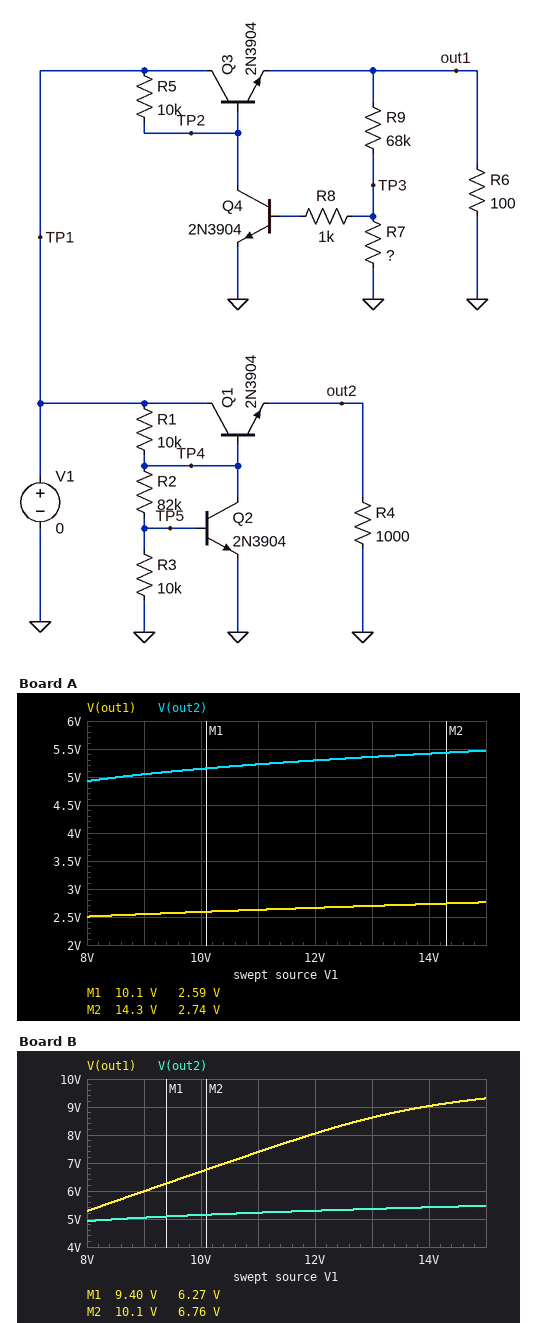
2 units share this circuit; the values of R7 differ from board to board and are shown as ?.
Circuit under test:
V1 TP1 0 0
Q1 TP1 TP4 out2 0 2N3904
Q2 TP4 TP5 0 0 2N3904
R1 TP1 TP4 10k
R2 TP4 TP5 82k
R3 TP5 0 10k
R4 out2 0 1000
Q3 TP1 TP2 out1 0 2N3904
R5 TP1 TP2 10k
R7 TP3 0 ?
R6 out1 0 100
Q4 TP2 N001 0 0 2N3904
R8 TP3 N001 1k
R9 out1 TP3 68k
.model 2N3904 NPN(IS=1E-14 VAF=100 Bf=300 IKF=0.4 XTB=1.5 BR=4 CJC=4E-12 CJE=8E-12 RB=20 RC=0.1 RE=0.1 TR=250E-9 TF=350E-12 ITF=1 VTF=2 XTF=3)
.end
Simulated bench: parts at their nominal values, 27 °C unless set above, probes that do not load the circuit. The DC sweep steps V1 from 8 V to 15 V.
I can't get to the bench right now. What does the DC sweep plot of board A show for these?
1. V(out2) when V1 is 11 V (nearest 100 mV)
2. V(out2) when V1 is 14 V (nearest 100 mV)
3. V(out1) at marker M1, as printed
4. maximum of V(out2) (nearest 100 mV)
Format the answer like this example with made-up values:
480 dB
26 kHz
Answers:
5.2 V
5.4 V
2.59 V
5.5 V
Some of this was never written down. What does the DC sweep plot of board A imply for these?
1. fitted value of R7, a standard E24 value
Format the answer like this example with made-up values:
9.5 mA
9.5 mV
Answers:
24 kΩ
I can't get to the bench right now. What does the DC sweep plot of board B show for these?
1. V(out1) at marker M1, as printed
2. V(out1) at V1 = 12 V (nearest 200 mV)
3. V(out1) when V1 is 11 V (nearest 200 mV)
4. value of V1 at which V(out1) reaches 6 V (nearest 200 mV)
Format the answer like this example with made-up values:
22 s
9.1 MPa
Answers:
6.27 V
8.0 V
7.4 V
9.0 V
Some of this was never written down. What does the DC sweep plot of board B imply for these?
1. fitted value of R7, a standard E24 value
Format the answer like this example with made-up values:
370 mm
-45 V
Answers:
4.7 kΩ
